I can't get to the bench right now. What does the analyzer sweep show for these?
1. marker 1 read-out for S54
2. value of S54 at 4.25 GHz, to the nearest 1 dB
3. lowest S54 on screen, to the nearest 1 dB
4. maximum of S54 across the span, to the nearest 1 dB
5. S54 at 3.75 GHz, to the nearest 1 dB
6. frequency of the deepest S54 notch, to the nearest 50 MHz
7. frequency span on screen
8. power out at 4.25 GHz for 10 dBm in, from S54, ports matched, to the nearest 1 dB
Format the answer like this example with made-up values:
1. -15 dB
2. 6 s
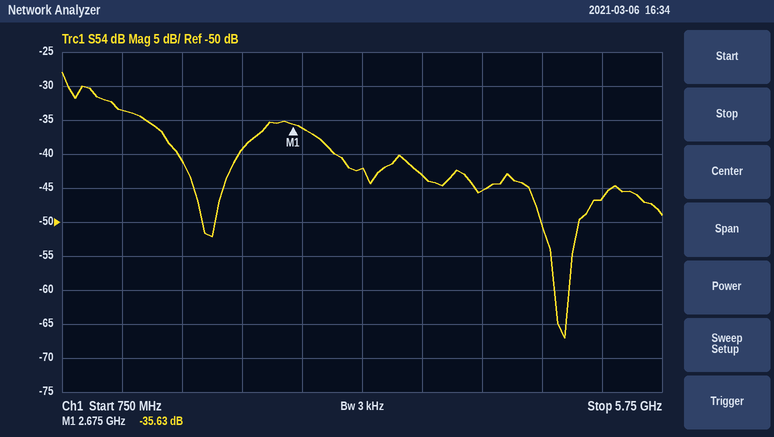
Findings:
1. -35.63 dB
2. -45 dB
3. -67 dB
4. -28 dB
5. -43 dB
6. 4.95 GHz
7. 5 GHz
8. -35 dBm
